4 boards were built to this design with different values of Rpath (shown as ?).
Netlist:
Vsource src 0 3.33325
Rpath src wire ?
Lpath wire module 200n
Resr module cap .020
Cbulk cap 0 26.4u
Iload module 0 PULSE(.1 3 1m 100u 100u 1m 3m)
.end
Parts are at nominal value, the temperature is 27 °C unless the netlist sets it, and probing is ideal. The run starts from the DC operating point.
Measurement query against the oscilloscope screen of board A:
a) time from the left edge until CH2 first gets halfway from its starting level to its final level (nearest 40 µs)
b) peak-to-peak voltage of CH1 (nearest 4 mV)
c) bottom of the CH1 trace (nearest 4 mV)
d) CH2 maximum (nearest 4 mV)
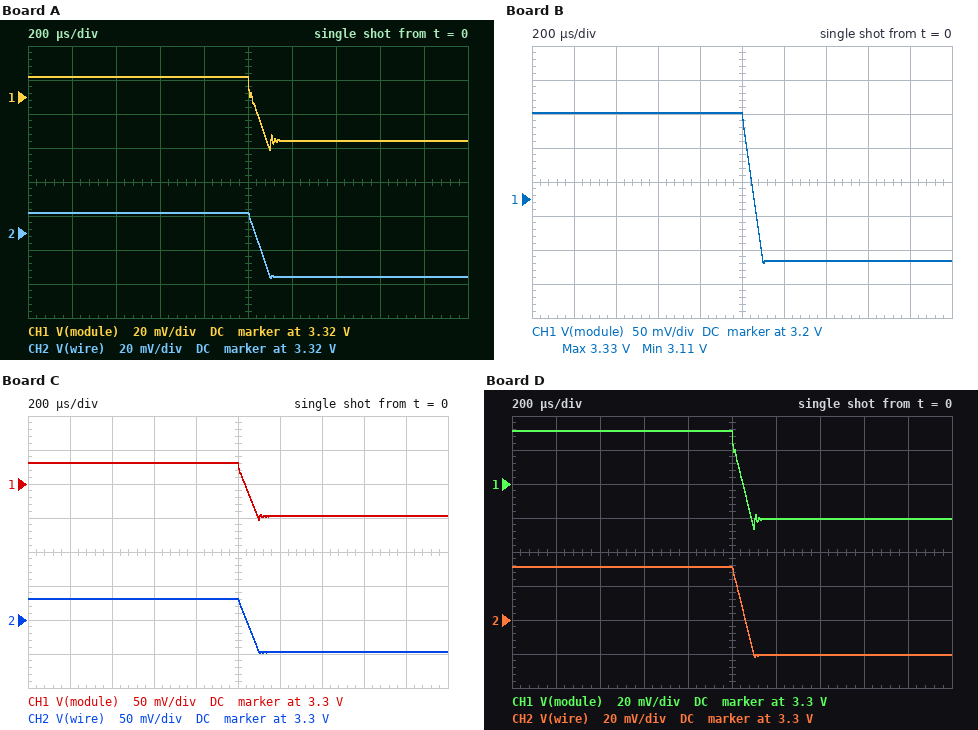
1.04 ms
44 mV
3.288 V
3.332 V
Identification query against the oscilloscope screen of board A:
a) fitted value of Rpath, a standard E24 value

0.013 Ω
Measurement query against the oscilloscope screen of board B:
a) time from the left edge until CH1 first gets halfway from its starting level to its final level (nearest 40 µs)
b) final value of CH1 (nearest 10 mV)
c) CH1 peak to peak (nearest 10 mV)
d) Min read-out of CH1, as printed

1.04 ms
3.11 V
220 mV
3.11 V
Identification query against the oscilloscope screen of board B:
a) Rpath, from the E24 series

0.075 Ω
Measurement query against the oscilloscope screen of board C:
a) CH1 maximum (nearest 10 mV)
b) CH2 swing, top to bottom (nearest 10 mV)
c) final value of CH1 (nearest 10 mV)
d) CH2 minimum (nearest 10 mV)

3.33 V
80 mV
3.25 V
3.25 V
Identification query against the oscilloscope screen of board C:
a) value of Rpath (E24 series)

0.027 Ω
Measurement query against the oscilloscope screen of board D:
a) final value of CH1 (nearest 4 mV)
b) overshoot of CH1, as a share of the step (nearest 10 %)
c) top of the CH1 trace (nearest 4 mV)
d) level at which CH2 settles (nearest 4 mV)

3.280 V
10 %
3.332 V
3.280 V
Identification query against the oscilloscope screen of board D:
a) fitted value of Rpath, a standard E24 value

0.018 Ω
